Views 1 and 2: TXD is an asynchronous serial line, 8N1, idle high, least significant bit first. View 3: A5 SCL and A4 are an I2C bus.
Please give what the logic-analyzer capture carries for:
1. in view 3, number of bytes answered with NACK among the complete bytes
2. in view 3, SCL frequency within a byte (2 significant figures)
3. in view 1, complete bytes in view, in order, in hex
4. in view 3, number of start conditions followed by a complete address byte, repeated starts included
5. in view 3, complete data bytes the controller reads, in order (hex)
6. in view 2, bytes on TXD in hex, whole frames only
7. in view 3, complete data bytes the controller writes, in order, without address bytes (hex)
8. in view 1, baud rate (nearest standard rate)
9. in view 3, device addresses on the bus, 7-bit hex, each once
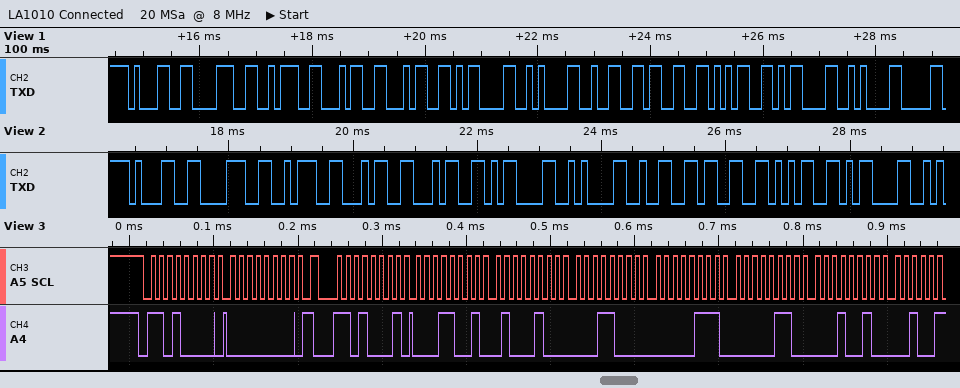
0
100 kHz
0x31 0x38 0x3A 0x34 0x34 0x0D 0x0A 0x32 0x33 0x35 0x0D 0x0A
2
19 44 18 07 06 12
31 38 3A 34 34 0D 0A 32 33 35 0D
00
9600 baud
0x68
